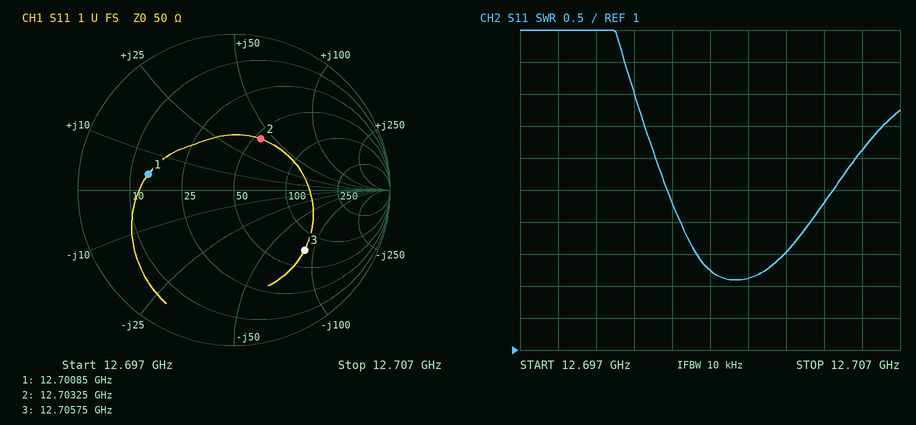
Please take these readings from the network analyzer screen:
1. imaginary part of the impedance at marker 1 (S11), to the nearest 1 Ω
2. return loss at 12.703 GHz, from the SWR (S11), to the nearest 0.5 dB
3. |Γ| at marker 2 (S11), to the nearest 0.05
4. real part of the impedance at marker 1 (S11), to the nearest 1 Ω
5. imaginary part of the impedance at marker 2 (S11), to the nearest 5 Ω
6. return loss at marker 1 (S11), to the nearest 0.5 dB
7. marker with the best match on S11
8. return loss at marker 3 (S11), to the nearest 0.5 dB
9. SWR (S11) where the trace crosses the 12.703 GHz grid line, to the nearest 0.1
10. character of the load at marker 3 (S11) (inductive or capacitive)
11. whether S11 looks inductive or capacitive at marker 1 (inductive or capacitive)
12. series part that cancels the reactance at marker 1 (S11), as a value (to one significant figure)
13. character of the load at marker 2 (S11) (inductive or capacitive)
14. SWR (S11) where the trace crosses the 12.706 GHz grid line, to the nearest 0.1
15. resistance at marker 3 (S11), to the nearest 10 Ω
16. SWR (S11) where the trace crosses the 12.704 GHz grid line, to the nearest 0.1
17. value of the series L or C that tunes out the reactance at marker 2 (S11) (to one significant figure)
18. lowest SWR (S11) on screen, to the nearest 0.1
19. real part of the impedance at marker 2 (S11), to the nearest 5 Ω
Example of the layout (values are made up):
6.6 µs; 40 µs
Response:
+4 Ω; 9.0 dB; 0.35; 14 Ω; +40 Ω; 5.0 dB; marker 2; 4.5 dB; 2.1; capacitive; inductive; 3 pF; inductive; 4.1; 70 Ω; 2.5; 300 fF; 2.1; 55 Ω
